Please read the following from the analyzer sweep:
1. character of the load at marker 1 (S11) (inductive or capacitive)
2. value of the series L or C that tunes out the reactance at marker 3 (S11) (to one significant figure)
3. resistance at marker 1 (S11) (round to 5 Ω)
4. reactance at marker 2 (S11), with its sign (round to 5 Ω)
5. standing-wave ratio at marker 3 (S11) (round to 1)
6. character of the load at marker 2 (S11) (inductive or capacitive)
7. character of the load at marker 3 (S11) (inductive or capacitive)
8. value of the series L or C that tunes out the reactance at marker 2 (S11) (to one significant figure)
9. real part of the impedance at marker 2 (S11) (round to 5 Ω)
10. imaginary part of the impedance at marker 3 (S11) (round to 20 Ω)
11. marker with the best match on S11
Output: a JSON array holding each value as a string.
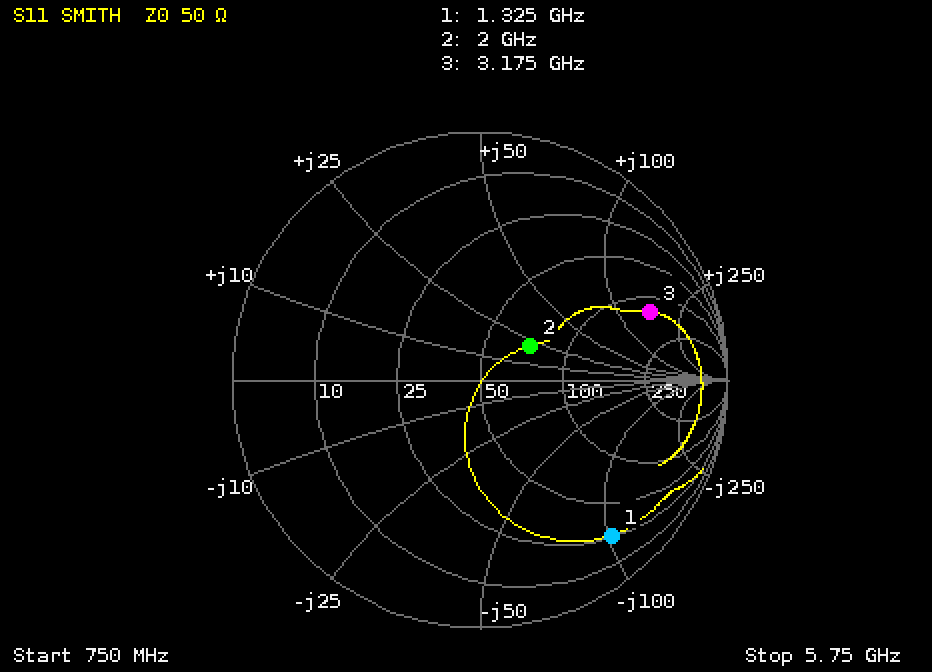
["capacitive", "300 fF", "25 Ω", "+20 Ω", "7", "inductive", "inductive", "4 pF", "70 Ω", "+160 Ω", "marker 2"]
